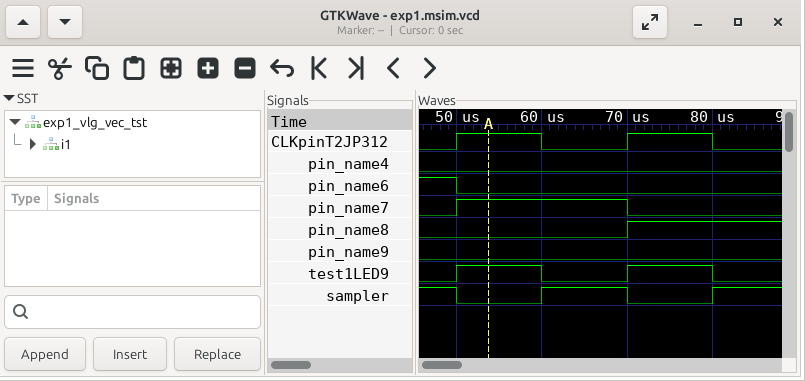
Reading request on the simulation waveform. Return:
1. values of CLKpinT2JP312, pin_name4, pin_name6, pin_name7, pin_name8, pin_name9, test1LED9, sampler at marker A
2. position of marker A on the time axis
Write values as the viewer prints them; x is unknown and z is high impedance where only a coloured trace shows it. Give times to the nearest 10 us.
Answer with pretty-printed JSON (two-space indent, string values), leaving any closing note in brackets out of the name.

{
  "values of CLKpinT2JP312, pin_name4, pin_name6, pin_name7, pin_name8, pin_name9, test1LED9, sampler at marker A": "CLKpinT2JP312=1, pin_name4=0, pin_name6=0, pin_name7=1, pin_name8=0, pin_name9=0, test1LED9=1, sampler=0",
  "position of marker A on the time axis": "50 us"
}
